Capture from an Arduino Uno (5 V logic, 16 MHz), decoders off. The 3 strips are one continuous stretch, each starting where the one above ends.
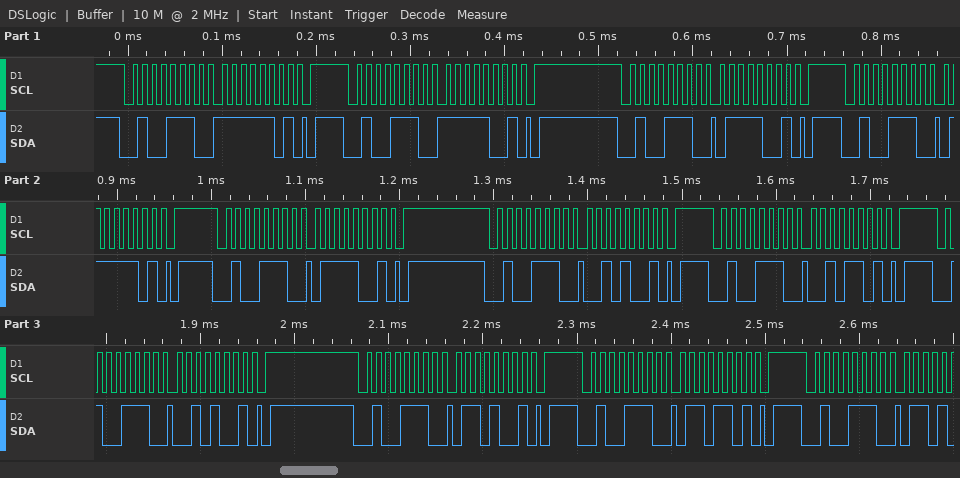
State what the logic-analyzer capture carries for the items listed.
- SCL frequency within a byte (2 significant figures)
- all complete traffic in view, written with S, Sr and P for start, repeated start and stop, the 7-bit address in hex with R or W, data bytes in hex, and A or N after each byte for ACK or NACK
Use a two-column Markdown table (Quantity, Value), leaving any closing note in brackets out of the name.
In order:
| Quantity | Value |
|---|---|
| SCL frequency within a byte | 100 kHz |
| all complete traffic in view, written with S, Sr and P for start, repeated start and stop, the 7-bit address in hex with R or W, data bytes in hex, and A or N after each byte for ACK or NACK | S 27W A FD A P S 27W A F9 A P S 27W A 79 A P S 27W A 7D A P S 27W A 79 A P S 27W A 29 A P S 27W A 2D A P S 27W A 29 A P S 27W A 69 A P S 27W A 6D A P S 27W A |
